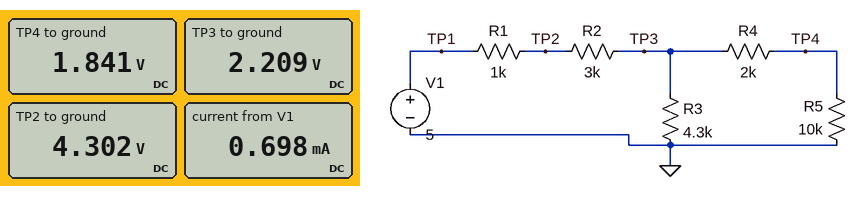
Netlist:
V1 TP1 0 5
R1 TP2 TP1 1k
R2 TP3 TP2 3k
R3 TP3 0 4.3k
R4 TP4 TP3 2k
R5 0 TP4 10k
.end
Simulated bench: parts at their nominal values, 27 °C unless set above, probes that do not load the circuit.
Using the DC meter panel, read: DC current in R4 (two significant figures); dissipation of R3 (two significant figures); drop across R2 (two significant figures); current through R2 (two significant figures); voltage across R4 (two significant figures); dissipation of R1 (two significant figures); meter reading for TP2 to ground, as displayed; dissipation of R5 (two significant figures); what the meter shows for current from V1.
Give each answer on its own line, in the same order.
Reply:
180 µA
1.1 mW
2.1 V
700 µA
370 mV
490 µW
4.302 V
340 µW
0.698 mA
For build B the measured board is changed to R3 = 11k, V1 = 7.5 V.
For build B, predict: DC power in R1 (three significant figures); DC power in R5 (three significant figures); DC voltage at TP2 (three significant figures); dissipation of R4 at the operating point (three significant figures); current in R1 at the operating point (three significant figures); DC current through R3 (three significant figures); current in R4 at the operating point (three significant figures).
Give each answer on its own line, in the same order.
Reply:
593 µW
1.36 mW
6.73 V
271 µW
770 µA
402 µA
368 µA
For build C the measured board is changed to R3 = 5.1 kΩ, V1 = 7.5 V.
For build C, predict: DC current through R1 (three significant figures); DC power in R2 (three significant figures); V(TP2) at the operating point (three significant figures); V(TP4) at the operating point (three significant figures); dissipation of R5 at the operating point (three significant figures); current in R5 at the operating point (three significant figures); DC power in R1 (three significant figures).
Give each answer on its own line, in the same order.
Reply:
990 µA
2.94 mW
6.51 V
2.95 V
871 µW
295 µA
979 µW
